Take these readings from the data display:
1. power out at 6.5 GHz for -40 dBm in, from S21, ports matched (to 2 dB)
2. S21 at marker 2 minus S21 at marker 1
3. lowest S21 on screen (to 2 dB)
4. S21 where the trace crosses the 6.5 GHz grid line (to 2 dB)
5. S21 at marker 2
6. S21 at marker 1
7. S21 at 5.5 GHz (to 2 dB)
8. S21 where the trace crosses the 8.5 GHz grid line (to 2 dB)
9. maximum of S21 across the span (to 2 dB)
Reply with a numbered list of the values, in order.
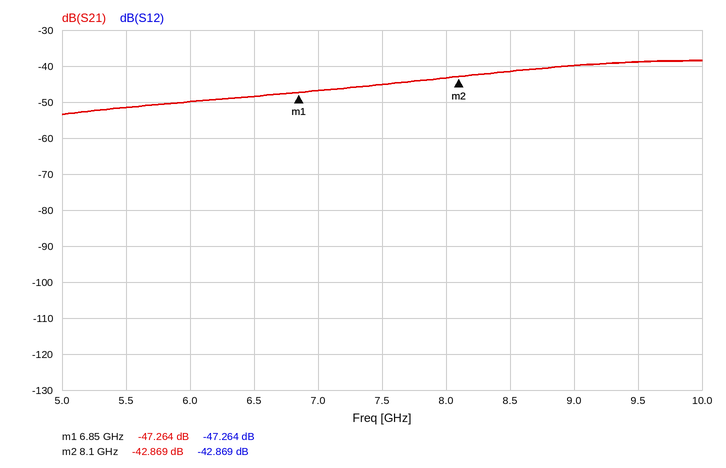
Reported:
1. -88 dBm
2. 4.395 dB
3. -54 dB
4. -48 dB
5. -42.869 dB
6. -47.264 dB
7. -52 dB
8. -42 dB
9. -38 dB
